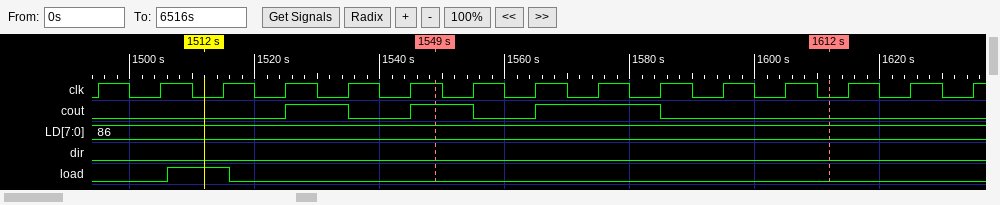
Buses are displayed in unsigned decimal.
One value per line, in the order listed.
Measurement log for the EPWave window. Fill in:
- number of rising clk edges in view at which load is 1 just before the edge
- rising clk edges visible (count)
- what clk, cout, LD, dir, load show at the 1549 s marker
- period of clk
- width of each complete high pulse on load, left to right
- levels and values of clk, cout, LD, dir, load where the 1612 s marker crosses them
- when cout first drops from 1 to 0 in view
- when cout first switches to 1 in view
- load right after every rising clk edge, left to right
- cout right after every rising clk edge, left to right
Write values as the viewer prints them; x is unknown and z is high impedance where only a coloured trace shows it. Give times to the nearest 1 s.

1
15
clk=1, cout=1, LD=86, dir=0, load=0
10 s
10 s
clk=0, cout=0, LD=86, dir=0, load=0
1535 s
1525 s
0 0 1 0 0 0 0 0 0 0 0 0 0 0 0
0 0 0 1 0 1 0 1 1 0 0 0 0 0 0
